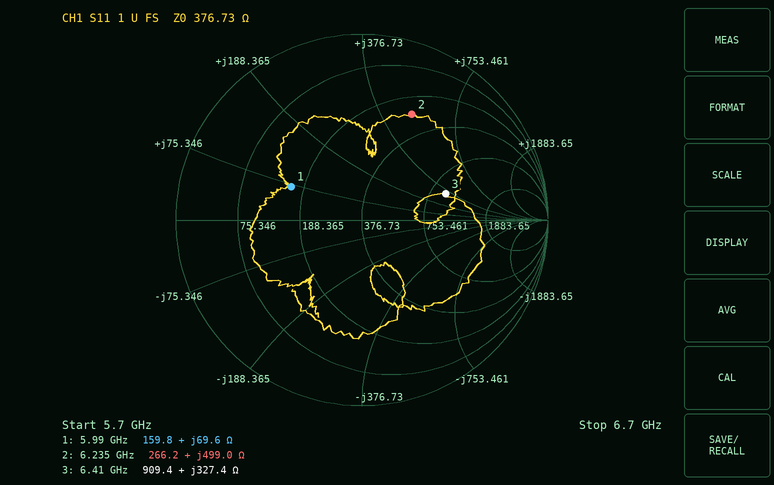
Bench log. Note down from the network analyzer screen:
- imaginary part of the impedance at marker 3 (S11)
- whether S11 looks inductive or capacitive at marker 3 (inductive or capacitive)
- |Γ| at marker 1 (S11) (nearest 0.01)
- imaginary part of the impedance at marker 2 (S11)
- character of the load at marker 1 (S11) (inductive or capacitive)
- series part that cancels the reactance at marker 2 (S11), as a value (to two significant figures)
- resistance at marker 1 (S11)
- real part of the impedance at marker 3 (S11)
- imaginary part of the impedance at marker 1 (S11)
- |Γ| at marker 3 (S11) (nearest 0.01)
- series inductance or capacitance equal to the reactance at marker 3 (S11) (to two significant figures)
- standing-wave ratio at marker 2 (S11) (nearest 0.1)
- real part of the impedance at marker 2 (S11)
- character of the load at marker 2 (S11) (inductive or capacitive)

+327.4 Ω
inductive
0.42
+499.0 Ω
inductive
51 fF
159.8 Ω
909.4 Ω
+69.6 Ω
0.47
8.1 nH
4.4
266.2 Ω
inductive
